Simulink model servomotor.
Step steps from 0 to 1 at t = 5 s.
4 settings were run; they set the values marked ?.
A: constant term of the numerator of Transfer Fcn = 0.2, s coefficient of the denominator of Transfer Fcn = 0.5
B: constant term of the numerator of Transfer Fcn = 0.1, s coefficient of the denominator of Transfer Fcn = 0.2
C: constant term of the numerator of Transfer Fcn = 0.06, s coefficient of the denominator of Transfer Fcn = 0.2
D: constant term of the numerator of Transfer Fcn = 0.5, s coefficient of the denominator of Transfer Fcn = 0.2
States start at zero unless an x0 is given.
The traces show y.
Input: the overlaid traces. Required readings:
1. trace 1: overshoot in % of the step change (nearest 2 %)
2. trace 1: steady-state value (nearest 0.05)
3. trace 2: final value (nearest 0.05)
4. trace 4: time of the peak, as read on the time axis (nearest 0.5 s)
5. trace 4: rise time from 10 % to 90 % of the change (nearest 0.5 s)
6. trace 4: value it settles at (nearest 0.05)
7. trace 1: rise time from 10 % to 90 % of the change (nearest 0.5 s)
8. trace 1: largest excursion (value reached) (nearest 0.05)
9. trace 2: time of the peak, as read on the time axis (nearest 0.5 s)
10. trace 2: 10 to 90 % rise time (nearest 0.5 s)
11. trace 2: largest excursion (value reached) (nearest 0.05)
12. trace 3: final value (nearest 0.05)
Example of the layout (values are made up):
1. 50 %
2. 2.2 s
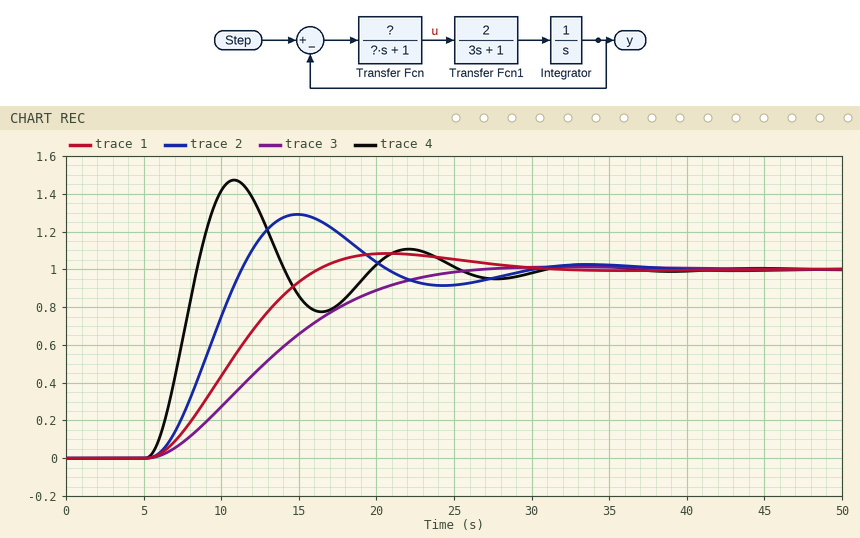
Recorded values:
1. 8 %
2. 1.00
3. 1.00
4. 11.0 s
5. 2.0 s
6. 1.00
7. 7.5 s
8. 1.10
9. 15.0 s
10. 4.0 s
11. 1.30
12. 1.00
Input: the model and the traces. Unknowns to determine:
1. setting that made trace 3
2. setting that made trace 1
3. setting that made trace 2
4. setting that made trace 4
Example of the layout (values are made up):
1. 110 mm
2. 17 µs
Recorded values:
1. C
2. B
3. A
4. D
